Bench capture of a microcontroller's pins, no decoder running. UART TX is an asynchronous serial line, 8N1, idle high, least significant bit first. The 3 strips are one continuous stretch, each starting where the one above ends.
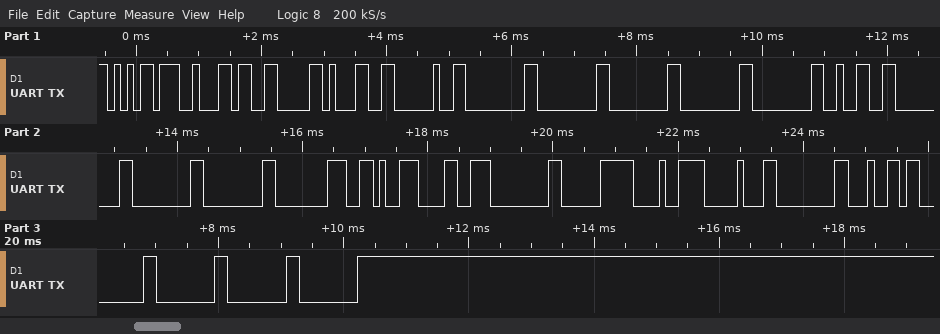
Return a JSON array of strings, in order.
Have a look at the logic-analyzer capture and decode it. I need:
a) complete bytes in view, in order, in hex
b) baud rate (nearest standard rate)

["0xB5 0x62 0x06 0x31 0x20 0x00 0x00 0x00 0x00 0x00 0x32 0x00 0x00 0x00 0x80 0x96 0x98 0x00 0xE0 0xC8 0x10 0x00 0x64 0x00 0x00 0x00 0x00", "9600 baud"]
